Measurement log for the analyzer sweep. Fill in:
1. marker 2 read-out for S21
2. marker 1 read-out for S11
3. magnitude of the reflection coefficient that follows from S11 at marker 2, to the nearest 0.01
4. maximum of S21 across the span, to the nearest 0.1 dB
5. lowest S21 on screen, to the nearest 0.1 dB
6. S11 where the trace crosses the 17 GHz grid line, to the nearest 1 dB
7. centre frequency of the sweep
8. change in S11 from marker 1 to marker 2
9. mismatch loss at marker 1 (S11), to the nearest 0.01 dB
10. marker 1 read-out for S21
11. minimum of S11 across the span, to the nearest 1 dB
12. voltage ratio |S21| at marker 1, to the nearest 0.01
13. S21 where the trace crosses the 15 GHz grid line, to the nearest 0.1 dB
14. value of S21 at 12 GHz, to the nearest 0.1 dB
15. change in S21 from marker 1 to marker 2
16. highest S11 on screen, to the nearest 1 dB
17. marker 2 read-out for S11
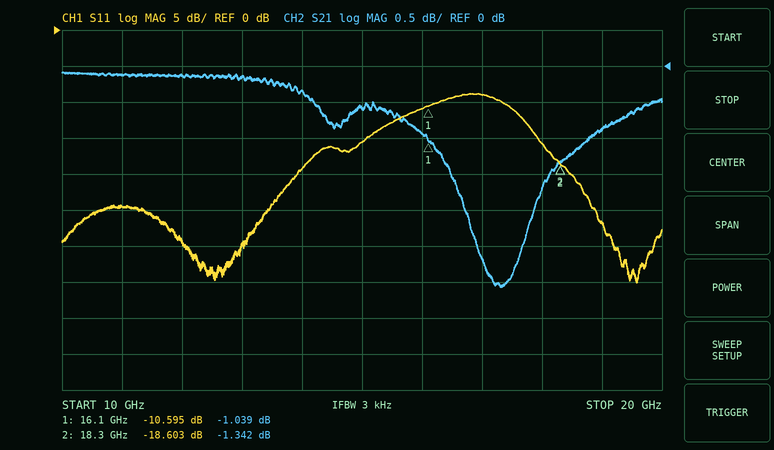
-1.342 dB
-10.595 dB
0.12
-0.1 dB
-3.1 dB
-9 dB
15 GHz
-8.008 dB
0.40 dB
-1.039 dB
-35 dB
0.89
-0.6 dB
-0.1 dB
-0.303 dB
-9 dB
-18.603 dB
